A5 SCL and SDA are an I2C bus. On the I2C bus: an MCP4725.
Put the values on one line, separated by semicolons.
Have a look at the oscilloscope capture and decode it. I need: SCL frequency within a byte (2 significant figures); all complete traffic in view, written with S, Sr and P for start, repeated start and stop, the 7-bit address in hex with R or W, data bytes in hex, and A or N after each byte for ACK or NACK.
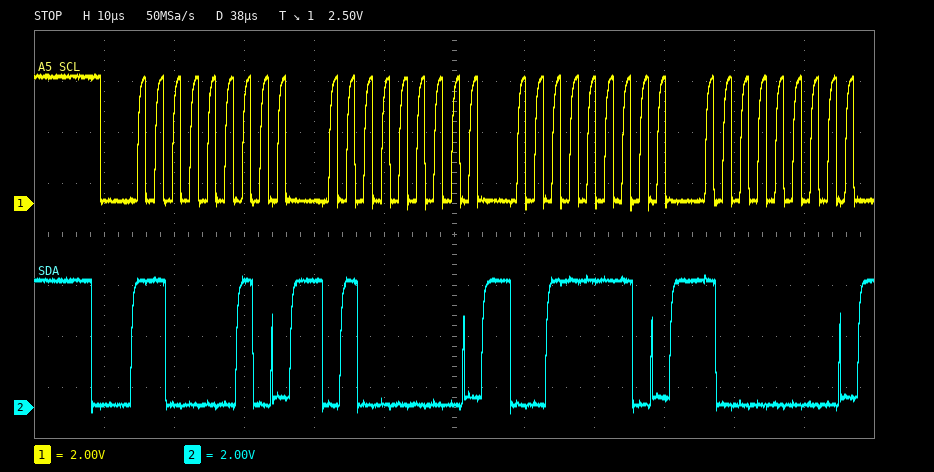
400 kHz; S 61W A 40 A 3E A 80 A
